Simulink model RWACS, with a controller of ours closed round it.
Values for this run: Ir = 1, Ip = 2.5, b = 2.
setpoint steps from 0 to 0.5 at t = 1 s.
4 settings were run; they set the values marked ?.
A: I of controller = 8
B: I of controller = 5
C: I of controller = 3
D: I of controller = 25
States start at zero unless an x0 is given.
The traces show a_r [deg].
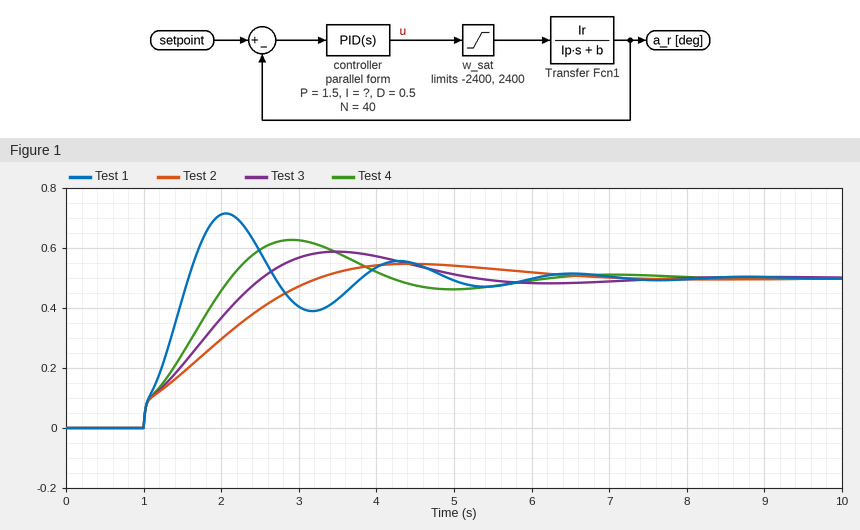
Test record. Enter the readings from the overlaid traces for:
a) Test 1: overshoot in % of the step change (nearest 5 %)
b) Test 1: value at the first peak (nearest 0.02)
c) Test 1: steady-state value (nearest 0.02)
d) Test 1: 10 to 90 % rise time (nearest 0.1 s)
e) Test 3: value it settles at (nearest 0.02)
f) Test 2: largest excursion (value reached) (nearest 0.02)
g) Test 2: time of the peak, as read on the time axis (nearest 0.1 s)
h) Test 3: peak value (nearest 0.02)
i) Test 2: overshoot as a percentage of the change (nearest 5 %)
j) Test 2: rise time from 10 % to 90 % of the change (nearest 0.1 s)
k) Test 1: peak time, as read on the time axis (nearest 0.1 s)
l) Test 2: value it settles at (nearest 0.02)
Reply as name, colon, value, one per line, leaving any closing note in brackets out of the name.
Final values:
Test 1: overshoot in % of the step change: 45 %
Test 1: value at the first peak: 0.72
Test 1: steady-state value: 0.50
Test 1: 10 to 90 % rise time: 0.5 s
Test 3: value it settles at: 0.50
Test 2: largest excursion (value reached): 0.54
Test 2: time of the peak, as read on the time axis: 4.4 s
Test 3: peak value: 0.58
Test 2: overshoot as a percentage of the change: 10 %
Test 2: rise time from 10 % to 90 % of the change: 1.8 s
Test 1: peak time, as read on the time axis: 2.1 s
Test 2: value it settles at: 0.50
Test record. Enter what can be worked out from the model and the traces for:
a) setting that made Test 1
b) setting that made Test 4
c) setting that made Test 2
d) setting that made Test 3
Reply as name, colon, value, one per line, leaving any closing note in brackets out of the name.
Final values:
setting that made Test 1: D
setting that made Test 4: A
setting that made Test 2: C
setting that made Test 3: B
